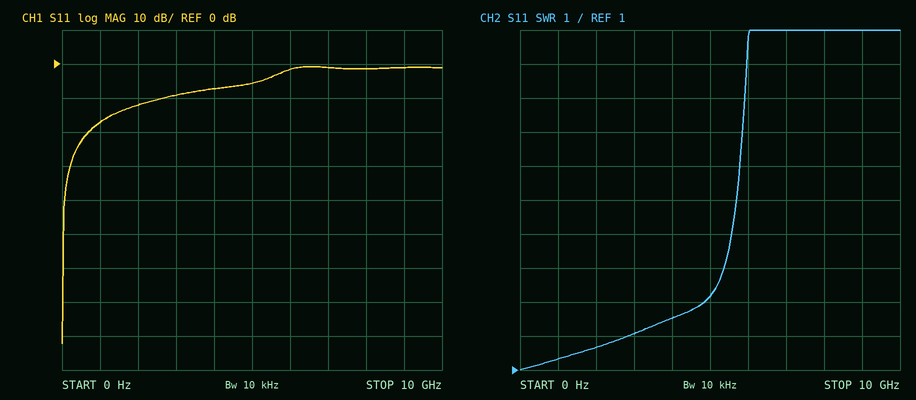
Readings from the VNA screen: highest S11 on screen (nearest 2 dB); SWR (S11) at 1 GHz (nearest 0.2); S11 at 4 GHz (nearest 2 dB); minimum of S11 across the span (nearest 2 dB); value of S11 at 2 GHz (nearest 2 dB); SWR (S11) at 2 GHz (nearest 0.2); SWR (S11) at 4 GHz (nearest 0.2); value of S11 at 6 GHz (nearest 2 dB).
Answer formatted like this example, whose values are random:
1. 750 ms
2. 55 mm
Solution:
1. 0 dB
2. 1.4
3. -8 dB
4. -82 dB
5. -12 dB
6. 1.6
7. 2.6
8. -2 dB
